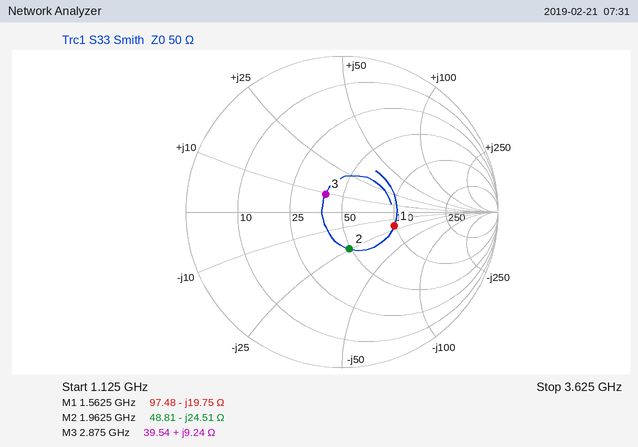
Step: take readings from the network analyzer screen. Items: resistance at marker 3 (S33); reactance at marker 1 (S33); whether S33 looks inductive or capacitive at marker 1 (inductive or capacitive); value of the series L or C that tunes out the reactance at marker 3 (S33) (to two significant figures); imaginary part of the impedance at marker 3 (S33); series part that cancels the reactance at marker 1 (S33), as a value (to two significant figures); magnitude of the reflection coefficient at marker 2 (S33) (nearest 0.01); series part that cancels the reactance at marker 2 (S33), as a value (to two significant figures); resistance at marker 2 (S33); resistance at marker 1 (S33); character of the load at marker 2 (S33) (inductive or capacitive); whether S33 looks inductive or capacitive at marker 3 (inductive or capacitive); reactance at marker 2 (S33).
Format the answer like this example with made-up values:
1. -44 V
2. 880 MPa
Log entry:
1. 39.54 Ω
2. -19.75 Ω
3. capacitive
4. 6.0 pF
5. +9.24 Ω
6. 2.0 nH
7. 0.24
8. 2.0 nH
9. 48.81 Ω
10. 97.48 Ω
11. capacitive
12. inductive
13. -24.51 Ω
